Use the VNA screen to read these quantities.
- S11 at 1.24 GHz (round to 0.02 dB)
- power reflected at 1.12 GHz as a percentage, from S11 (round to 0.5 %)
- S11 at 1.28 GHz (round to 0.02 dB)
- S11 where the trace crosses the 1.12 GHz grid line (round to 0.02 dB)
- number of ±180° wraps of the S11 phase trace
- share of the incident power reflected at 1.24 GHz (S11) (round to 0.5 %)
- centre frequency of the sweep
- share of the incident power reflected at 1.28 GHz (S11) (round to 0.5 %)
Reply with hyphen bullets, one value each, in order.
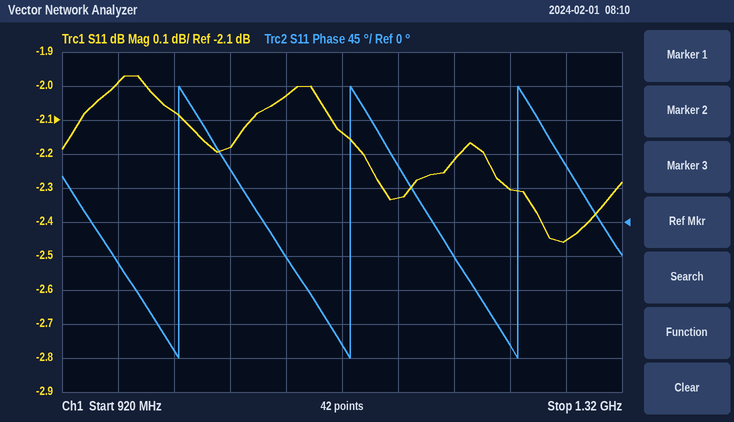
- -2.30 dB
- 61.0 %
- -2.46 dB
- -2.14 dB
- 3
- 59.0 %
- 1.12 GHz
- 57.0 %
